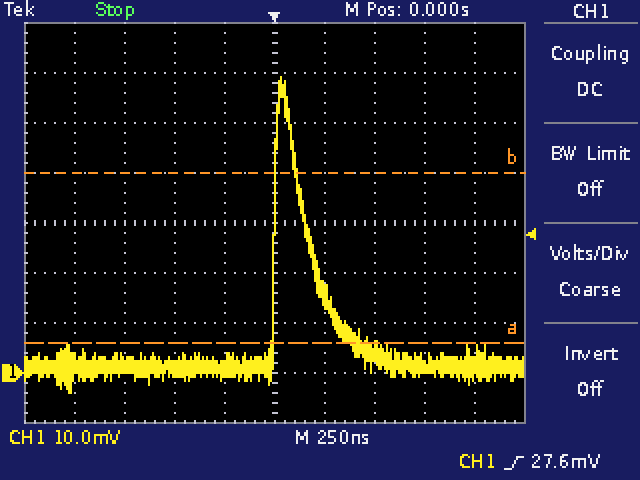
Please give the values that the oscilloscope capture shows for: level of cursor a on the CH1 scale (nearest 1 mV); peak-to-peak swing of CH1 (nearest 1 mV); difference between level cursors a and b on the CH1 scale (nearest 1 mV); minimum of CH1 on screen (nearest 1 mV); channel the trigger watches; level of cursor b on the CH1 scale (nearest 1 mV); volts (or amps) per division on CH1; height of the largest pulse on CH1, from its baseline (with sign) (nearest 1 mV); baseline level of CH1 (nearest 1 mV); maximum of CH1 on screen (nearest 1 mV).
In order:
6 mV
63 mV
34 mV
-4 mV
CH1
40 mV
10 mV
+58 mV
1 mV
59 mV
